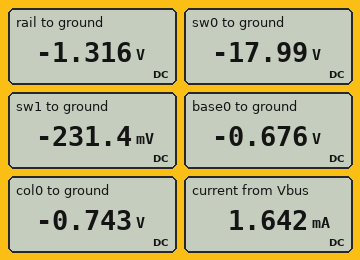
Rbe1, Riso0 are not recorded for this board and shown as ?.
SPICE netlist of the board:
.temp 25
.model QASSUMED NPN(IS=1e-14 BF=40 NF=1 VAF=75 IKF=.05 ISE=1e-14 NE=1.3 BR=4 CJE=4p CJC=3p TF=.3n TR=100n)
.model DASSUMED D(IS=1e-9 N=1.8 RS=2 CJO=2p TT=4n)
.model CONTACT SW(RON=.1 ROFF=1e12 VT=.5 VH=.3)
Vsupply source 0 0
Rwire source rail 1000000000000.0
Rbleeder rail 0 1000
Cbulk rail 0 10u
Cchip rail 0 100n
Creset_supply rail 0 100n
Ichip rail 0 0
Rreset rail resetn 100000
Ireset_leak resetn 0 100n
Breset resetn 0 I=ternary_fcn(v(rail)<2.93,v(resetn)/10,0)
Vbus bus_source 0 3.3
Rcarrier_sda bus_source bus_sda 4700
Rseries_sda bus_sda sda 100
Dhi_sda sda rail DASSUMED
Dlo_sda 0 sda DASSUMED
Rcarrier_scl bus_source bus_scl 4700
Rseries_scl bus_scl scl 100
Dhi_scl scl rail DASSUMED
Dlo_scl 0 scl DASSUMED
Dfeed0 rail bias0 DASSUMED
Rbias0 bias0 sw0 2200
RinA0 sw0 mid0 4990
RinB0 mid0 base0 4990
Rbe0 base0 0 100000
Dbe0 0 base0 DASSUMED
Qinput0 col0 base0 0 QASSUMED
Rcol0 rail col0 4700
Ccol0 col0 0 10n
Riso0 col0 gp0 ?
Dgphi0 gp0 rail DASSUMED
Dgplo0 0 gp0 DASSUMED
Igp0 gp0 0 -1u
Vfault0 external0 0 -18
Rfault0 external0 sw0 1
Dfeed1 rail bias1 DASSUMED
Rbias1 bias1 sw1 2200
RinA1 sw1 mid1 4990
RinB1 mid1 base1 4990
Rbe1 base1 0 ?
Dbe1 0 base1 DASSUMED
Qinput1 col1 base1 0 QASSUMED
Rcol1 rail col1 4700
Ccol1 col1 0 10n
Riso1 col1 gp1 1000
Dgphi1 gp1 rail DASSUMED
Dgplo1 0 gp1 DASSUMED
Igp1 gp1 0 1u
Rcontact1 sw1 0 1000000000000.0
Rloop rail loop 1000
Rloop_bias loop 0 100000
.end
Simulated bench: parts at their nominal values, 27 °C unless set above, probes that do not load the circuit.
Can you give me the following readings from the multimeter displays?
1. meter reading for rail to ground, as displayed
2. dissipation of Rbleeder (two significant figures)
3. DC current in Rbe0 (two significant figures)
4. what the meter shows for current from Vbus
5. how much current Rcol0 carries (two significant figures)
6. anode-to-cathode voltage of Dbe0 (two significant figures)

-1.316 V
1.7 mW
6.8 µA
1.642 mA
120 µA
680 mV
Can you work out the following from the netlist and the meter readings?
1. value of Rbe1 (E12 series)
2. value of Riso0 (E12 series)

120 kΩ
680 Ω
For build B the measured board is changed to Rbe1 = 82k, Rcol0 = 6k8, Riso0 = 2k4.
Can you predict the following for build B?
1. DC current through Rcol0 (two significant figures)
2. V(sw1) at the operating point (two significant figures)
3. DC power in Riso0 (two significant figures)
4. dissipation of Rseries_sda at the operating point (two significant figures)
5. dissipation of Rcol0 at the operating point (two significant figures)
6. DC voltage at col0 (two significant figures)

71 µA
-220 mV
12 µW
67 µW
35 µW
-830 mV
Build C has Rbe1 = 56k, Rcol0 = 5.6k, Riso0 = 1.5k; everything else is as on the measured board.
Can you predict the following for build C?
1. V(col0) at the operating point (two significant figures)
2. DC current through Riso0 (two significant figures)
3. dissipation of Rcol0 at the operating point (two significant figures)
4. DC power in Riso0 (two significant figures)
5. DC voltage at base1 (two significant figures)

-800 mV
92 µA
48 µW
13 µW
-210 mV
